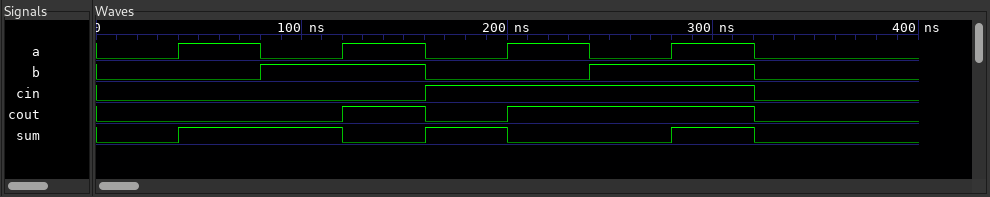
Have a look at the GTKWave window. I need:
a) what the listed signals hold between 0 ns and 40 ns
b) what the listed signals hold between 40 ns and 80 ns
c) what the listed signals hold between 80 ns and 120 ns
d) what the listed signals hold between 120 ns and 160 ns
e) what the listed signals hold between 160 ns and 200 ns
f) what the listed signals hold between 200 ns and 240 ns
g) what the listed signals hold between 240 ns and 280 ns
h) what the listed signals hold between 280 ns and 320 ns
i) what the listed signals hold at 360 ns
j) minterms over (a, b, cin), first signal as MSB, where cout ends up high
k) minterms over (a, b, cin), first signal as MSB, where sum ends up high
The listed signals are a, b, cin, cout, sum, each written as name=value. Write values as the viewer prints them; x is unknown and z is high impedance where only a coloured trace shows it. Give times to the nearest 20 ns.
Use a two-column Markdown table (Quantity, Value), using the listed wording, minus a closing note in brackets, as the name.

| Quantity | Value |
|---|---|
| what the listed signals hold between 0 ns and 40 ns | a=0, b=0, cin=0, cout=0, sum=0 |
| what the listed signals hold between 40 ns and 80 ns | a=1, b=0, cin=0, cout=0, sum=1 |
| what the listed signals hold between 80 ns and 120 ns | a=0, b=1, cin=0, cout=0, sum=1 |
| what the listed signals hold between 120 ns and 160 ns | a=1, b=1, cin=0, cout=1, sum=0 |
| what the listed signals hold between 160 ns and 200 ns | a=0, b=0, cin=1, cout=0, sum=1 |
| what the listed signals hold between 200 ns and 240 ns | a=1, b=0, cin=1, cout=1, sum=0 |
| what the listed signals hold between 240 ns and 280 ns | a=0, b=1, cin=1, cout=1, sum=0 |
| what the listed signals hold between 280 ns and 320 ns | a=1, b=1, cin=1, cout=1, sum=1 |
| what the listed signals hold at 360 ns | a=0, b=0, cin=0, cout=0, sum=0 |
| minterms over (a, b, cin), first signal as MSB, where cout ends up high | 3, 5, 6, 7 |
| minterms over (a, b, cin), first signal as MSB, where sum ends up high | 1, 2, 4, 7 |
